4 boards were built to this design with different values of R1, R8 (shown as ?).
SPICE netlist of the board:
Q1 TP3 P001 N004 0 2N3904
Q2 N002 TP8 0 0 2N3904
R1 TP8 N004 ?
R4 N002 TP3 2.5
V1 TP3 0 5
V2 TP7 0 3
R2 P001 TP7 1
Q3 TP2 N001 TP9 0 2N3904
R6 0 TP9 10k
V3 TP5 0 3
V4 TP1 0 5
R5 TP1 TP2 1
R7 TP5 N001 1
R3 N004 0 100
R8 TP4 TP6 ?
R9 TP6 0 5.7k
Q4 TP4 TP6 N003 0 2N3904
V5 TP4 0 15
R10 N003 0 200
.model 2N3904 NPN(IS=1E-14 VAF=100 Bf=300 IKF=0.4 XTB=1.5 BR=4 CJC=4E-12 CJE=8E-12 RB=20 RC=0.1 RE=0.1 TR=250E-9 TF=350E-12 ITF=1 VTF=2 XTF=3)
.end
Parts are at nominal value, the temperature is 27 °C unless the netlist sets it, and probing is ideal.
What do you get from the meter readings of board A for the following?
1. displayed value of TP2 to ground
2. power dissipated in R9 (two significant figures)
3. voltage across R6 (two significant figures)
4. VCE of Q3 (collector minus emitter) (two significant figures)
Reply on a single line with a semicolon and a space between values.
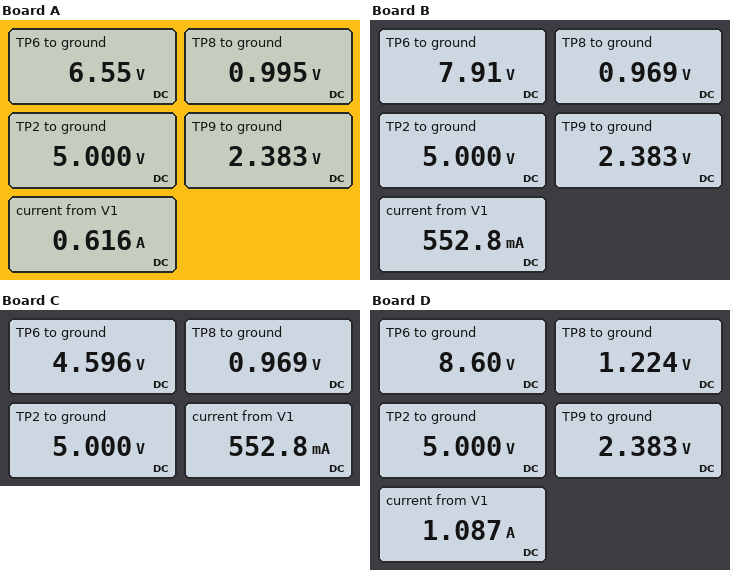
5.000 V; 7.5 mW; 2.4 V; 2.6 V
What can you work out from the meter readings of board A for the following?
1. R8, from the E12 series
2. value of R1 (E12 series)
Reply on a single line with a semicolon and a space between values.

6.8 kΩ; 270 Ω
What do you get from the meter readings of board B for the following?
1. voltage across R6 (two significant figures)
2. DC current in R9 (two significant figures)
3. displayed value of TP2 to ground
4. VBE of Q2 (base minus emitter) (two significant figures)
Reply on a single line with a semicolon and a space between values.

2.4 V; 1.4 mA; 5.000 V; 970 mV
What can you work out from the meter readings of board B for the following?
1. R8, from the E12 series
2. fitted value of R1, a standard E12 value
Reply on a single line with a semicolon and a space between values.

4.7 kΩ; 330 Ω
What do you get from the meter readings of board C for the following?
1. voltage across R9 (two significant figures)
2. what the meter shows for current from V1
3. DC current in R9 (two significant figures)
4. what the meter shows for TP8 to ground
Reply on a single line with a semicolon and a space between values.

4.6 V; 552.8 mA; 810 µA; 0.969 V
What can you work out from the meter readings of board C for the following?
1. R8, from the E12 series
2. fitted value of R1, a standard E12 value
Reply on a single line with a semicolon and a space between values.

12 kΩ; 330 Ω
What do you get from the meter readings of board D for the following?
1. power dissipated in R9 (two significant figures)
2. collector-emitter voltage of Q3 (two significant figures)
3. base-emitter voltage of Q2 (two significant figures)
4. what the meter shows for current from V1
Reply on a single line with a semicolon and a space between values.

13 mW; 2.6 V; 1.2 V; 1.087 A
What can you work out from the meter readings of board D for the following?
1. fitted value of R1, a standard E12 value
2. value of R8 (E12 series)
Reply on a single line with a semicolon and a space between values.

82 Ω; 3.9 kΩ
